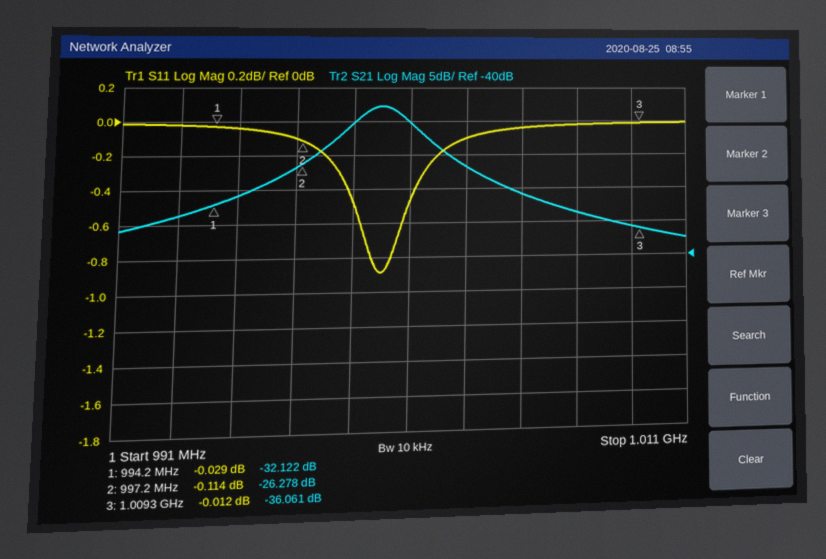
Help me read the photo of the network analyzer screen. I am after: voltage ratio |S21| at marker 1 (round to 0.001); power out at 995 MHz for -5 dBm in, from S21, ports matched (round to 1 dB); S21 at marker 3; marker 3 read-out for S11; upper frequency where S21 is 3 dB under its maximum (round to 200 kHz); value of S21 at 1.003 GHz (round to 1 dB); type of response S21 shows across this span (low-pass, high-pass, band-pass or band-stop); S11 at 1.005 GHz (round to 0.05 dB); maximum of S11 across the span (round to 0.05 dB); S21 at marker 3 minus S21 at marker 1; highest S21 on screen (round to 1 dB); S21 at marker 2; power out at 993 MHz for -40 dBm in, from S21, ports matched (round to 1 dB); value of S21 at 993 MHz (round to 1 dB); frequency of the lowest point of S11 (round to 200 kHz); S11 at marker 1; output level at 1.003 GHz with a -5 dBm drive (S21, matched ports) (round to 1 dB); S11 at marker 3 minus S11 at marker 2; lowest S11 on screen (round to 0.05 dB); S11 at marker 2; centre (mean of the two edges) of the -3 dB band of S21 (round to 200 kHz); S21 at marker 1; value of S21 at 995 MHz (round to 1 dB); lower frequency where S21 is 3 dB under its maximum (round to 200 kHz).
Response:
0.025
-36 dBm
-36.061 dB
-0.012 dB
1.0012 GHz
-27 dB
band-pass
-0.05 dB
0.00 dB
-3.939 dB
-18 dB
-26.278 dB
-74 dBm
-34 dB
1.0000 GHz
-0.029 dB
-32 dBm
0.102 dB
-0.90 dB
-0.114 dB
1.0000 GHz
-32.122 dB
-31 dB
998.8 MHz
